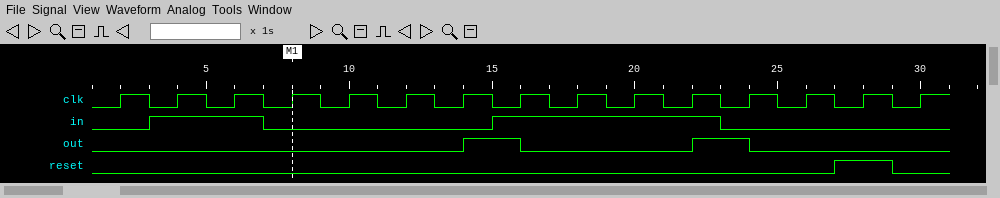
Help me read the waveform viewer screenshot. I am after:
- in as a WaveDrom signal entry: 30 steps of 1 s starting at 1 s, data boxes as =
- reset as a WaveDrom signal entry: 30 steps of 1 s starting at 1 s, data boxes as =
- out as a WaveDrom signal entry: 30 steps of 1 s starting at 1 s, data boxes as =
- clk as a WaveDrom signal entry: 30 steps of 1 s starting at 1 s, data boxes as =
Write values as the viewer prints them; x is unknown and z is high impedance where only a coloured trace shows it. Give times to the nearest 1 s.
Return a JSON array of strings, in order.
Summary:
["{name: 'in', wave: '0.1...0.......1.......0.......'}", "{name: 'reset', wave: '0.........................1.0.'}", "{name: 'out', wave: '0............1.0.....1.0......'}", "{name: 'clk', wave: '010101010101010101010101010101'}"]
